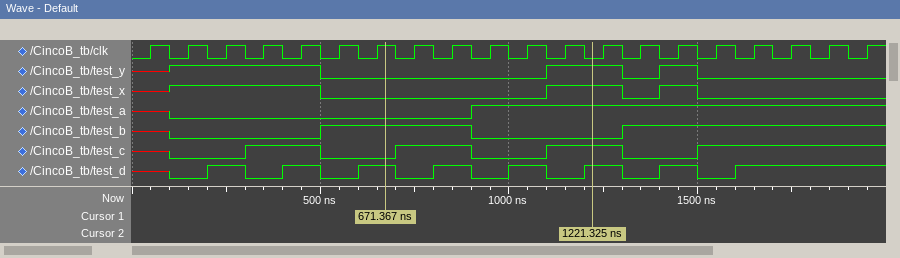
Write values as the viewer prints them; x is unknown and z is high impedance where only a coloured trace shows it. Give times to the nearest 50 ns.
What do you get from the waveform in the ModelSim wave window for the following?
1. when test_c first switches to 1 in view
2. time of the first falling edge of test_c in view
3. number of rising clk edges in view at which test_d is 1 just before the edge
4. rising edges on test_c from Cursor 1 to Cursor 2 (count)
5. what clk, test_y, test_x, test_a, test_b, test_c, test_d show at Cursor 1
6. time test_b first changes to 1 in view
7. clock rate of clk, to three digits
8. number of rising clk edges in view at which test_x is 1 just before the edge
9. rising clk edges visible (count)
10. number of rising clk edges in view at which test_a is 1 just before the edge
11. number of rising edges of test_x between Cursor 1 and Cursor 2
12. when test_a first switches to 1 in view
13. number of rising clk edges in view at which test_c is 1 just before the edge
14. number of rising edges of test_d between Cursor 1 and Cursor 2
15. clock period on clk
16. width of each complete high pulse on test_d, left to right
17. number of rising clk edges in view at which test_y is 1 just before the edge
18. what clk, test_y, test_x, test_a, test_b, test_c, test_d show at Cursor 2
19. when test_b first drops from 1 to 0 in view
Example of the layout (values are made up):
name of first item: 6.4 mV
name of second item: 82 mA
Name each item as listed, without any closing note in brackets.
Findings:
when test_c first switches to 1 in view: 300 ns
time of the first falling edge of test_c in view: 500 ns
number of rising clk edges in view at which test_d is 1 just before the edge: 11
rising edges on test_c from Cursor 1 to Cursor 2: 2
what clk, test_y, test_x, test_a, test_b, test_c, test_d show at Cursor 1: clk=1, test_y=0, test_x=0, test_a=0, test_b=1, test_c=0, test_d=1
time test_b first changes to 1 in view: 500 ns
clock rate of clk, to three digits: 10.0 MHz
number of rising clk edges in view at which test_x is 1 just before the edge: 7
rising clk edges visible: 20
number of rising clk edges in view at which test_a is 1 just before the edge: 11
number of rising edges of test_x between Cursor 1 and Cursor 2: 1
when test_a first switches to 1 in view: 900 ns
number of rising clk edges in view at which test_c is 1 just before the edge: 11
number of rising edges of test_d between Cursor 1 and Cursor 2: 3
clock period on clk: 100 ns
width of each complete high pulse on test_d, left to right: 100 ns, 100 ns, 100 ns, 100 ns, 100 ns, 100 ns, 100 ns
number of rising clk edges in view at which test_y is 1 just before the edge: 7
what clk, test_y, test_x, test_a, test_b, test_c, test_d show at Cursor 2: clk=0, test_y=1, test_x=1, test_a=1, test_b=0, test_c=1, test_d=1
when test_b first drops from 1 to 0 in view: 900 ns
